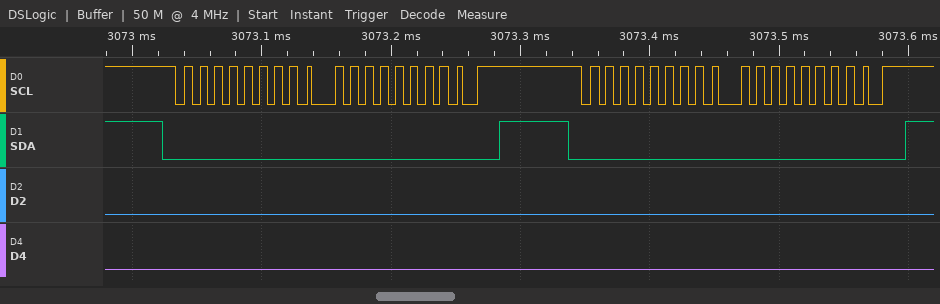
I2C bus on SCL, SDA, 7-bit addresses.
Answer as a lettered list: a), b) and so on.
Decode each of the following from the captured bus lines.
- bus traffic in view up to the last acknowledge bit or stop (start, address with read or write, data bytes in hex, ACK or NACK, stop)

a) start, address 00 write ACK, 00 ACK, stop, start, address 00 write ACK, 00 ACK, stop
